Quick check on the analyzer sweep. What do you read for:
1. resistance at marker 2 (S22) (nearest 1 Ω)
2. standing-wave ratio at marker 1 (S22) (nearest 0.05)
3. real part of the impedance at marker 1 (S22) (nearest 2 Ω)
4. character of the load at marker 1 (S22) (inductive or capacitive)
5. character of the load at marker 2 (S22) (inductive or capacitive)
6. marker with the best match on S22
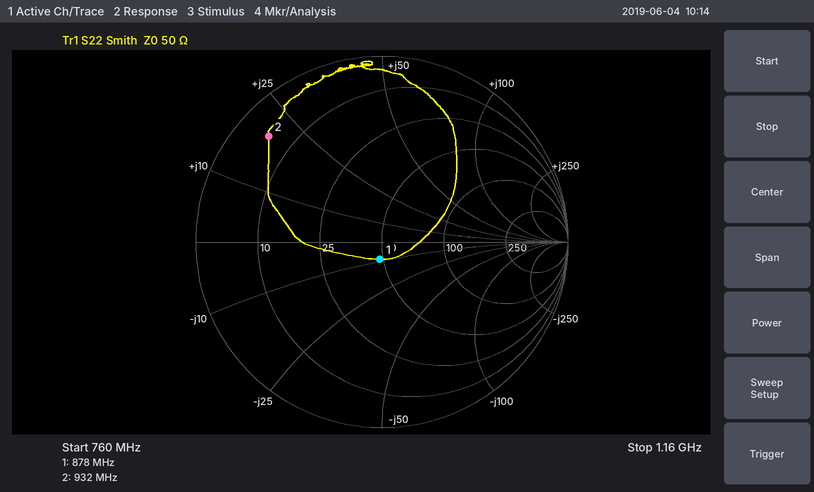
5 Ω
1.20
48 Ω
capacitive
inductive
marker 1
